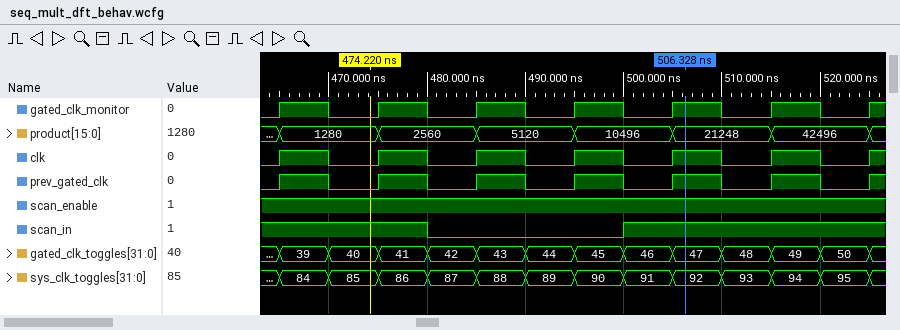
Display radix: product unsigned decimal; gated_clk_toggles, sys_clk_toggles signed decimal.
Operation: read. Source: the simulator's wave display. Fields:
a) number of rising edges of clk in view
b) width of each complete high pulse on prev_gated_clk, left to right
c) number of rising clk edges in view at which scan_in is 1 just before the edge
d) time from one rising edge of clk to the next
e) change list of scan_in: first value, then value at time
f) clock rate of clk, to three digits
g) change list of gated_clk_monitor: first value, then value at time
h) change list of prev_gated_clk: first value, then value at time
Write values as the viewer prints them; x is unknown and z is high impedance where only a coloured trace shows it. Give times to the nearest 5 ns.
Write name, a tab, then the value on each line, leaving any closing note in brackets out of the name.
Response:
number of rising edges of clk in view	7
width of each complete high pulse on prev_gated_clk, left to right	5 ns, 5 ns, 5 ns, 5 ns, 5 ns, 5 ns
number of rising clk edges in view at which scan_in is 1 just before the edge	5
time from one rising edge of clk to the next	10 ns
change list of scan_in: first value, then value at time	1, 0 at 480 ns, 1 at 500 ns
clock rate of clk, to three digits	100 MHz
change list of gated_clk_monitor: first value, then value at time	0, 1 at 465 ns, 0 at 470 ns, 1 at 475 ns, 0 at 480 ns, 1 at 485 ns, 0 at 490 ns, 1 at 495 ns, 0 at 500 ns, 1 at 505 ns, 0 at 510 ns, 1 at 515 ns, 0 at 520 ns, 1 at 525 ns
change list of prev_gated_clk: first value, then value at time	0, 1 at 465 ns, 0 at 470 ns, 1 at 475 ns, 0 at 480 ns, 1 at 485 ns, 0 at 490 ns, 1 at 495 ns, 0 at 500 ns, 1 at 505 ns, 0 at 510 ns, 1 at 515 ns, 0 at 520 ns, 1 at 525 ns
